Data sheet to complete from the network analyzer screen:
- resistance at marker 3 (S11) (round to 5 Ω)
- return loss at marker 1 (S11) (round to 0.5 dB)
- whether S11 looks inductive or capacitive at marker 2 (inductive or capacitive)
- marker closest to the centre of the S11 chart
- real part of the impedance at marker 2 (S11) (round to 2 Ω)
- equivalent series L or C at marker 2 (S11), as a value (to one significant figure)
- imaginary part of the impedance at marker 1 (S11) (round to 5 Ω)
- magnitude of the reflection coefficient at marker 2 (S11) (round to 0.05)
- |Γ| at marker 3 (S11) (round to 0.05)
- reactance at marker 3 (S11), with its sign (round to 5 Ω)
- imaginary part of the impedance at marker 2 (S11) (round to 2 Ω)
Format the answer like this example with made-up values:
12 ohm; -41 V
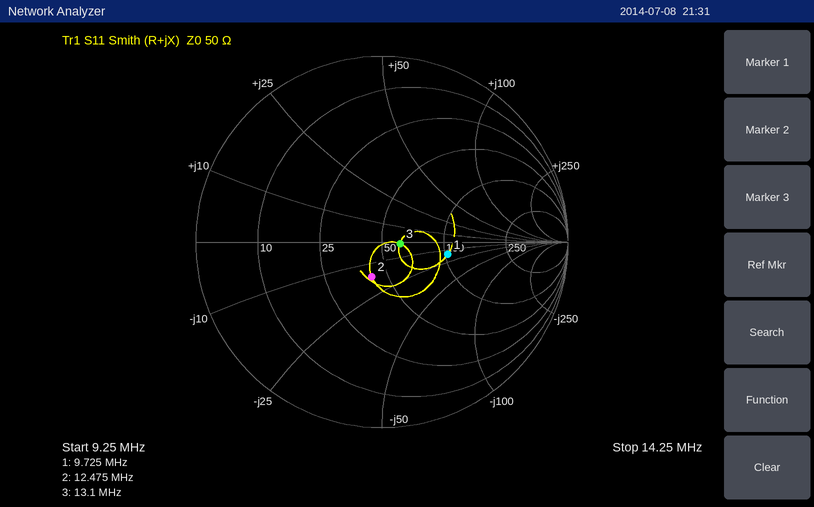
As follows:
60 Ω; 9.0 dB; capacitive; marker 3; 42 Ω; 800 pF; -15 Ω; 0.20; 0.10; 0 Ω; -16 Ω
